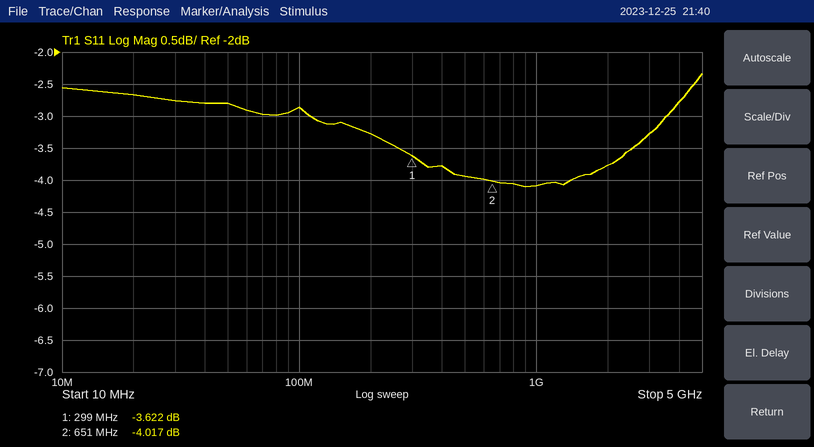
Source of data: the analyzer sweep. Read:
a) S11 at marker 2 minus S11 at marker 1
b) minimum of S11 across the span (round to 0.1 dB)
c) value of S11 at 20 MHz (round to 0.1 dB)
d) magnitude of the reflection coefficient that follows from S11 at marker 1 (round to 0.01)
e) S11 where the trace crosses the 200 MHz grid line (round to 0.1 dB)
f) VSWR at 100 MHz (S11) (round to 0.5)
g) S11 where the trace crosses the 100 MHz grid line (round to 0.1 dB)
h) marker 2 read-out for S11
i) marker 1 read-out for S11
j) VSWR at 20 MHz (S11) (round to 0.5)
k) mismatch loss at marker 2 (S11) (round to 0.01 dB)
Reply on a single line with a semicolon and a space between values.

-0.395 dB; -4.1 dB; -2.7 dB; 0.66; -3.3 dB; 6.0; -2.9 dB; -4.017 dB; -3.622 dB; 6.5; 2.19 dB
